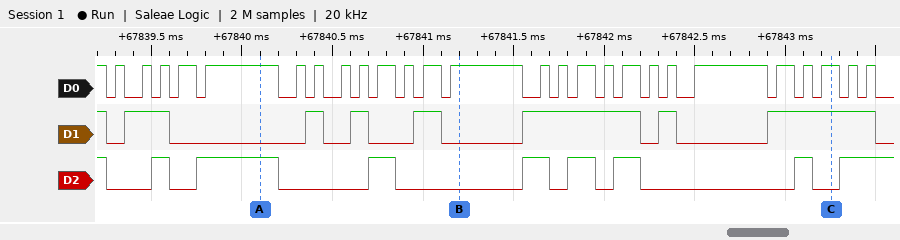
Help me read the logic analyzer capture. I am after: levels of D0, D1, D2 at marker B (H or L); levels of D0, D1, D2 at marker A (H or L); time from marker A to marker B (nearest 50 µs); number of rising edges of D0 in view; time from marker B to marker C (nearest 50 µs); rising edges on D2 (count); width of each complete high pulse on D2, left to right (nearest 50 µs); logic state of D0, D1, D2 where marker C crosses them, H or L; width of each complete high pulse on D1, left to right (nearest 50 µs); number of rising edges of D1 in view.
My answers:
D0=H, D1=L, D2=L
D0=H, D1=L, D2=H
1100 µs
26
2050 µs
8
100 µs, 450 µs, 150 µs, 150 µs, 150 µs, 150 µs, 100 µs
D0=H, D1=H, D2=L
250 µs, 100 µs, 100 µs, 150 µs, 650 µs, 100 µs, 600 µs
7
